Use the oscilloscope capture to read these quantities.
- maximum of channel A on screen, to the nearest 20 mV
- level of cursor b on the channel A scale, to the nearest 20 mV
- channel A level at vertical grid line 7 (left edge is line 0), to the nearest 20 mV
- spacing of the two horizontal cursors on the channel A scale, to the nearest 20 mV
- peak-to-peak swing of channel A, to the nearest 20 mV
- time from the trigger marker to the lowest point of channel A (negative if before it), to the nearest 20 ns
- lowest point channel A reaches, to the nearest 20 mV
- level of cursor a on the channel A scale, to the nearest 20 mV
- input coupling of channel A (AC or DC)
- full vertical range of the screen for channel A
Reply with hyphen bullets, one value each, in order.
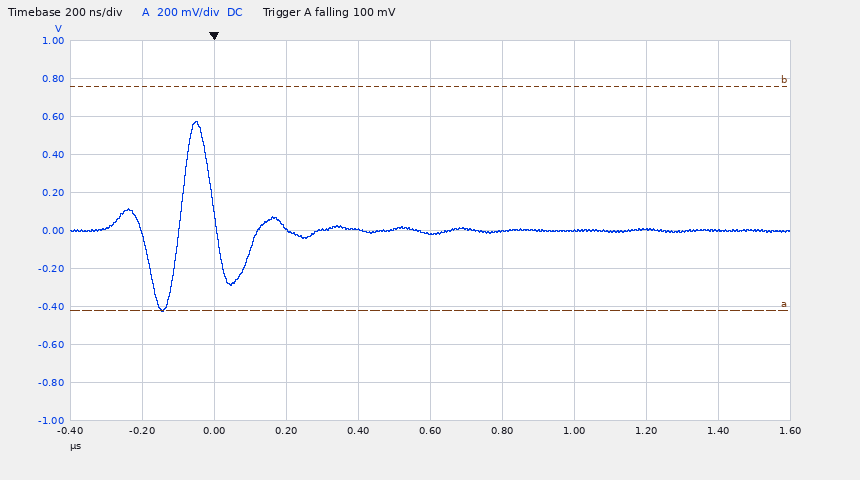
- 580 mV
- 760 mV
- 0 mV
- 1.18 V
- 1.00 V
- -140 ns
- -420 mV
- -420 mV
- DC
- 2 V
